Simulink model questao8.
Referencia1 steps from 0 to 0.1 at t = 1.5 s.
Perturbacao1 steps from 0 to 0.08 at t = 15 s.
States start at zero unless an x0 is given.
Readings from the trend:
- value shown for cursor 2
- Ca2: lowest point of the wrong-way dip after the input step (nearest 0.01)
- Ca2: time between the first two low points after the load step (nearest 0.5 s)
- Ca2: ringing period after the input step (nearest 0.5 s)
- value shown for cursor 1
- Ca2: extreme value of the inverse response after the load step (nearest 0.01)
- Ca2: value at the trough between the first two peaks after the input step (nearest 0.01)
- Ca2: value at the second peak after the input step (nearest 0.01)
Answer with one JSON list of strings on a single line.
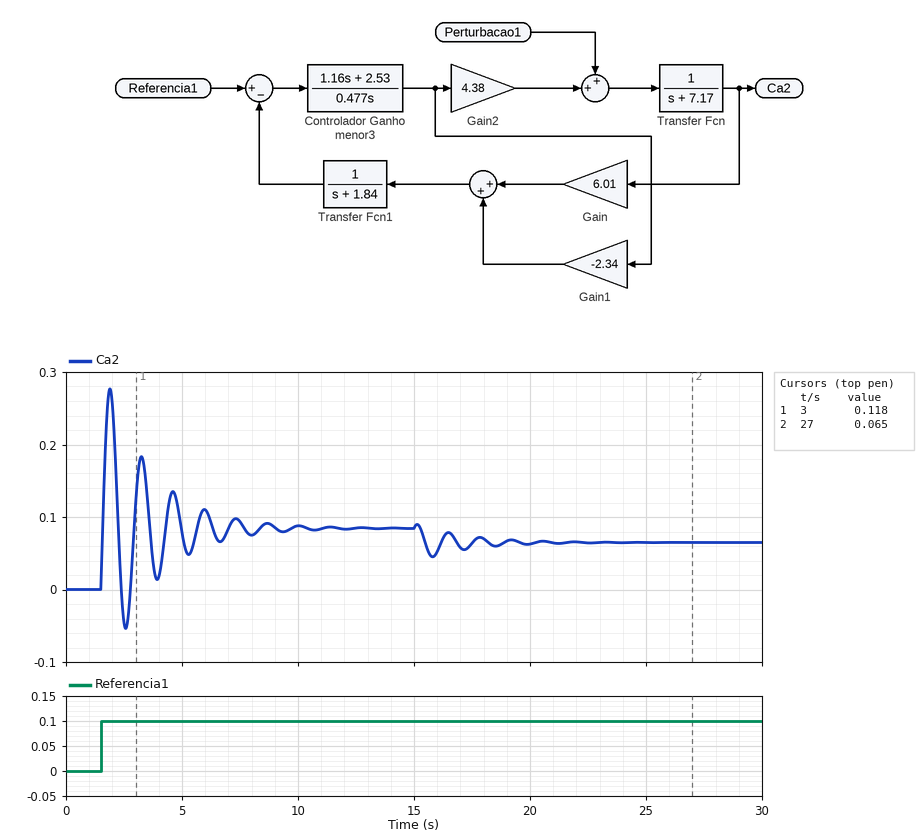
["0.065", "-0.05", "1.5 s", "1.5 s", "0.118", "0.09", "-0.05", "0.18"]
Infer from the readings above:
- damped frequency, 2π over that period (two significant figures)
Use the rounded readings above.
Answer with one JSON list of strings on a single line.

["4.2 rad/s"]
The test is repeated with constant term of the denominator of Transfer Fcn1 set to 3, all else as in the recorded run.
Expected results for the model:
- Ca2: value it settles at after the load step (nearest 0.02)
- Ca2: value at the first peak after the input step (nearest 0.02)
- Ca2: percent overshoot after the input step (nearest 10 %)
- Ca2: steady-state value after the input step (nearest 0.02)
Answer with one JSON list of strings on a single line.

["0.12", "0.26", "90 %", "0.14"]
